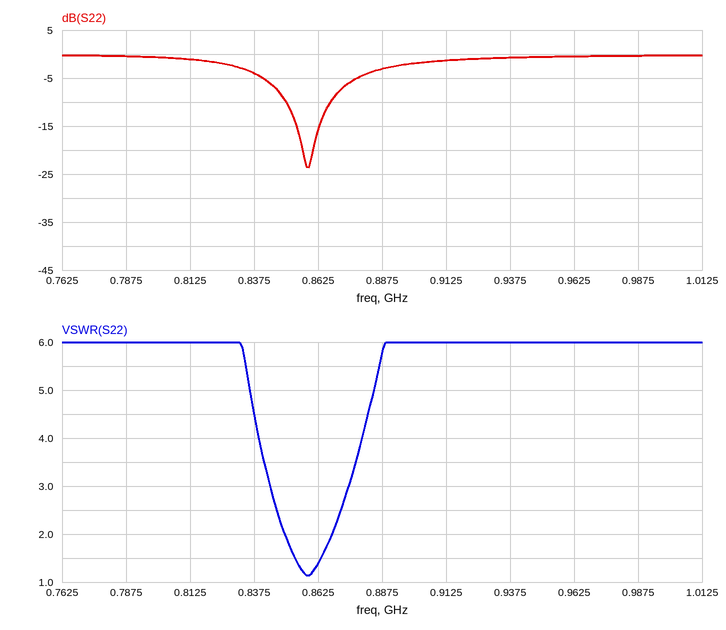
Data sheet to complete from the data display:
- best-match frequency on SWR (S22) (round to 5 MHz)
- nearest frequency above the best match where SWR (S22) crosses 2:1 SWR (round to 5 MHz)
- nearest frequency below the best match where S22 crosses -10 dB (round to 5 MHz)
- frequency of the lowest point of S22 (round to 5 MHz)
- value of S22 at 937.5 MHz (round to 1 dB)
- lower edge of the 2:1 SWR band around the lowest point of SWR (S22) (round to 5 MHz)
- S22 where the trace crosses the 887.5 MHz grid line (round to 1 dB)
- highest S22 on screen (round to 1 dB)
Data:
860 MHz
870 MHz
850 MHz
860 MHz
-1 dB
850 MHz
-3 dB
0 dB
